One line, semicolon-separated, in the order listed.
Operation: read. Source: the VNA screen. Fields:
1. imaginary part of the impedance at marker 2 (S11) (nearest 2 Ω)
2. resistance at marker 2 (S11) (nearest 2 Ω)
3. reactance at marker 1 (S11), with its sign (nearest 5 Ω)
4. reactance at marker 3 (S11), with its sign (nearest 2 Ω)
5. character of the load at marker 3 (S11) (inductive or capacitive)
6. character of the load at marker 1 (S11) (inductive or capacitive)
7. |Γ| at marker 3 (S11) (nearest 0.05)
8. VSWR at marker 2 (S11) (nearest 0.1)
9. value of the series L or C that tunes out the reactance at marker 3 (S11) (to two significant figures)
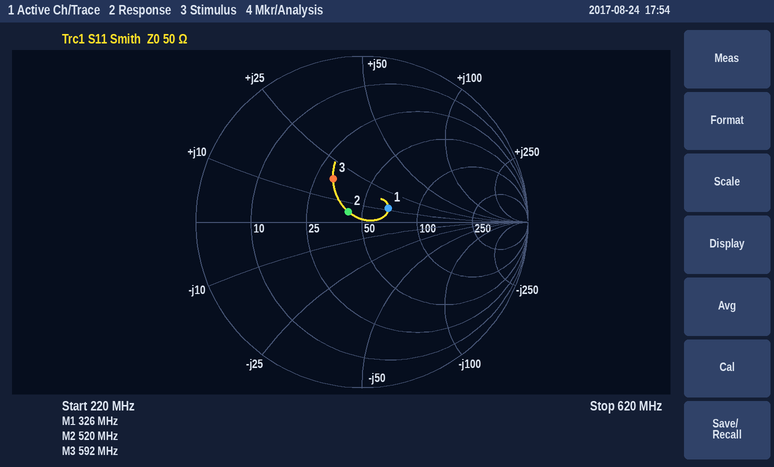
+6 Ω; 42 Ω; +10 Ω; +18 Ω; inductive; inductive; 0.30; 1.2; 15 pF
